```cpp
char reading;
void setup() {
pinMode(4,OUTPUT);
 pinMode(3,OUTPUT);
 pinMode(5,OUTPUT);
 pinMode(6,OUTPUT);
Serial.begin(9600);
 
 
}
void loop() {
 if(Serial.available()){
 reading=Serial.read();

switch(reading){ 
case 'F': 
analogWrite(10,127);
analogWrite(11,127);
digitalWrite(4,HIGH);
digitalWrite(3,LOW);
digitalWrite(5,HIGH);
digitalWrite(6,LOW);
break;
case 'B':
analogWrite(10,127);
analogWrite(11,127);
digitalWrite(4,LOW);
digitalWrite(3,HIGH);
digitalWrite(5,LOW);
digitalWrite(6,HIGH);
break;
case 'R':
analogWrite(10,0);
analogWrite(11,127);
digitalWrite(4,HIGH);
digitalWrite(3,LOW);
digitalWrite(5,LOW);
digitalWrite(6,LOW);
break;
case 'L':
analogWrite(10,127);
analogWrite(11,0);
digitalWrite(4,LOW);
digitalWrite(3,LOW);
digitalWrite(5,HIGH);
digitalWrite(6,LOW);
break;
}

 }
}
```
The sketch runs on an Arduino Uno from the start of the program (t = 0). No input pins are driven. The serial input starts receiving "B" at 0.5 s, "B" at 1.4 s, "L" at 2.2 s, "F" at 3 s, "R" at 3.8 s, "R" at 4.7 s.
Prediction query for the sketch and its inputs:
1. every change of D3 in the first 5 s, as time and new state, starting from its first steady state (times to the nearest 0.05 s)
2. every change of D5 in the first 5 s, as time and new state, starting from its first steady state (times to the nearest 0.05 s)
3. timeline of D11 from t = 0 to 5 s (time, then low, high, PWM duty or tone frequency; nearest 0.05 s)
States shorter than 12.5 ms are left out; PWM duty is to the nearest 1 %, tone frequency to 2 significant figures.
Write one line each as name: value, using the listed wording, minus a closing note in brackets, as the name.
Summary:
every change of D3 in the first 5 s, as time and new state, starting from its first steady state: 0 s low; 0.5 s high; 2.2 s low
every change of D5 in the first 5 s, as time and new state, starting from its first steady state: 0 s low; 2.2 s high; 3.8 s low
timeline of D11 from t = 0 to 5 s: 0.5 s PWM 50 %; 2.2 s low; 3 s PWM 50 %
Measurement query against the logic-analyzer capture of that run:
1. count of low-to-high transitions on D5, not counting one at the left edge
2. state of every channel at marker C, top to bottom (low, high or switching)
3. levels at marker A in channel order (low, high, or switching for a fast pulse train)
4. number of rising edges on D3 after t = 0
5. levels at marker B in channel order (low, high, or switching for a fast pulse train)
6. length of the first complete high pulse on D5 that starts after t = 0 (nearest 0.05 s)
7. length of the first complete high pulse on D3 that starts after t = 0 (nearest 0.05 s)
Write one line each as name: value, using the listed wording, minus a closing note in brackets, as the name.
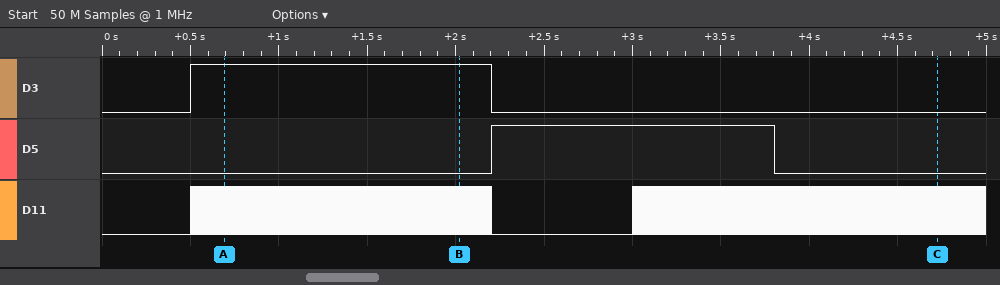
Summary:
count of low-to-high transitions on D5, not counting one at the left edge: 1
state of every channel at marker C, top to bottom: D3 low, D5 low, D11 switching
levels at marker A in channel order: D3 high, D5 low, D11 switching
number of rising edges on D3 after t = 0: 1
levels at marker B in channel order: D3 high, D5 low, D11 switching
length of the first complete high pulse on D5 that starts after t = 0: 1.60 s
length of the first complete high pulse on D3 that starts after t = 0: 1.70 s
